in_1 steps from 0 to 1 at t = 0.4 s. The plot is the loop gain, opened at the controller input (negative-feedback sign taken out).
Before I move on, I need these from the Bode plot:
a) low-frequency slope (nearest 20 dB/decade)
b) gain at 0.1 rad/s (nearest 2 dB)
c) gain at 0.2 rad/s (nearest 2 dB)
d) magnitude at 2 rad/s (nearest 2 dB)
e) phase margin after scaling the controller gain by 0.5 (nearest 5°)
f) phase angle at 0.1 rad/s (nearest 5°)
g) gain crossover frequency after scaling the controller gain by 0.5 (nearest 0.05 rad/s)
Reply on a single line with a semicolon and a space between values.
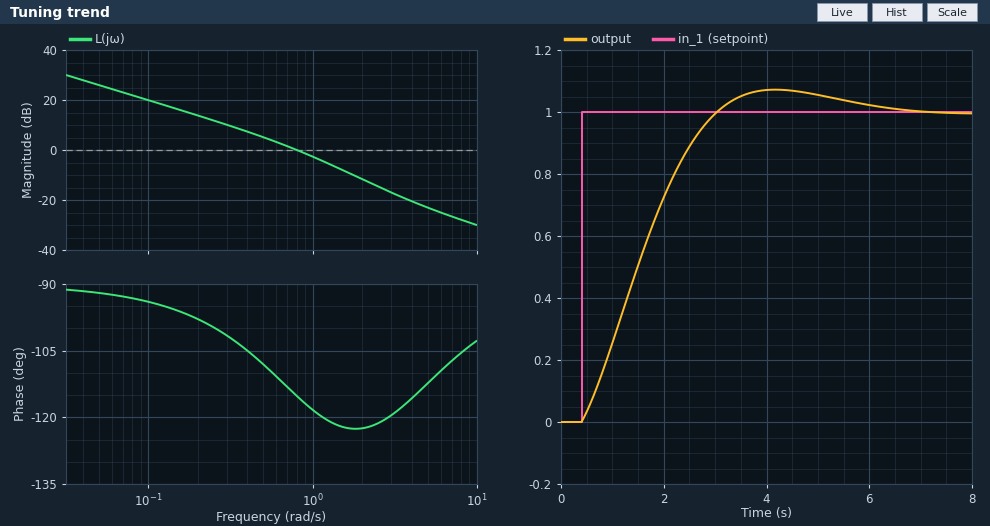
-20 dB/decade; 20 dB; 14 dB; -12 dB; 75°; -95°; 0.45 rad/s
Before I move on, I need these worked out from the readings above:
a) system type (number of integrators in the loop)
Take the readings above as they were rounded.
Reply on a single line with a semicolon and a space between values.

1
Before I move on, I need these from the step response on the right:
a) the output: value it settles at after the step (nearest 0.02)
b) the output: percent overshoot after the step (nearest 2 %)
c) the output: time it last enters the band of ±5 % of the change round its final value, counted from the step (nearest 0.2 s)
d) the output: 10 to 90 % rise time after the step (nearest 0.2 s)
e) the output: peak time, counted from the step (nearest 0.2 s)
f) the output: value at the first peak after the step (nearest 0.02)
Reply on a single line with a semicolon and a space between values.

1.00; 8 %; 4.8 s; 1.8 s; 3.8 s; 1.08
